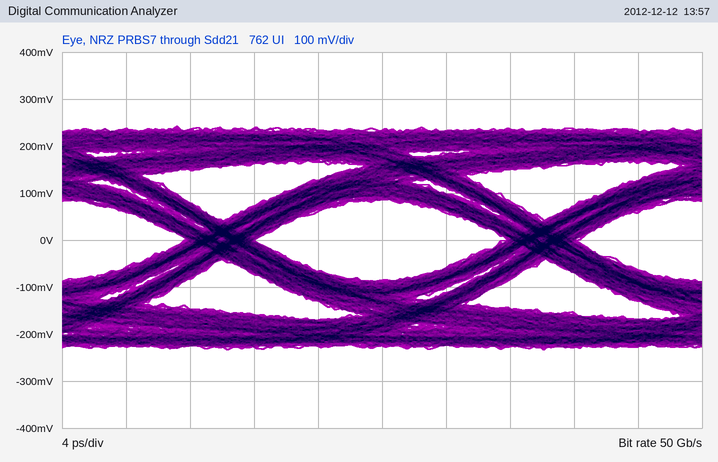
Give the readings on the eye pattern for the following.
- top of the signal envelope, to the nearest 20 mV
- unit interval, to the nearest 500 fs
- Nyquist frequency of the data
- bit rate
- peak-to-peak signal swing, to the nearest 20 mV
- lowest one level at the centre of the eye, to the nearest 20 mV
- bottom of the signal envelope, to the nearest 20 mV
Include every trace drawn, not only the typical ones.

240 mV
20.0 ps
25 GHz
50 Gb/s
480 mV
80 mV
-240 mV
